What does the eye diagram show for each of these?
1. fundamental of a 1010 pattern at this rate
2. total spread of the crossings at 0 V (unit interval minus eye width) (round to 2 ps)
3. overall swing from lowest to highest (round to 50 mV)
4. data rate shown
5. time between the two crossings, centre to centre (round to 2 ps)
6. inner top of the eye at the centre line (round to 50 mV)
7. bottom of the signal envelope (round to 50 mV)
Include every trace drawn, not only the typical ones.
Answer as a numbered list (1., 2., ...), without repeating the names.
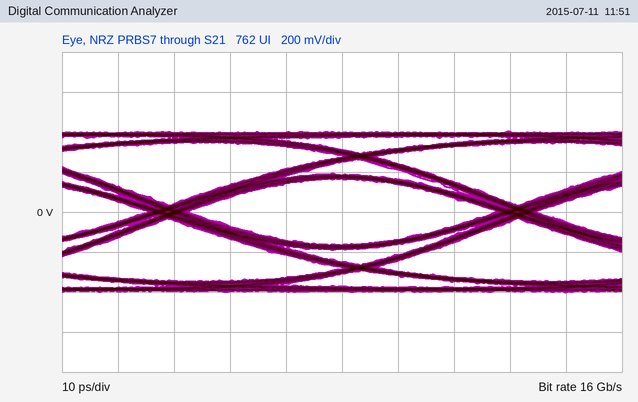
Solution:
1. 8 GHz
2. 8 ps
3. 800 mV
4. 16 Gb/s
5. 62 ps
6. 150 mV
7. -400 mV
